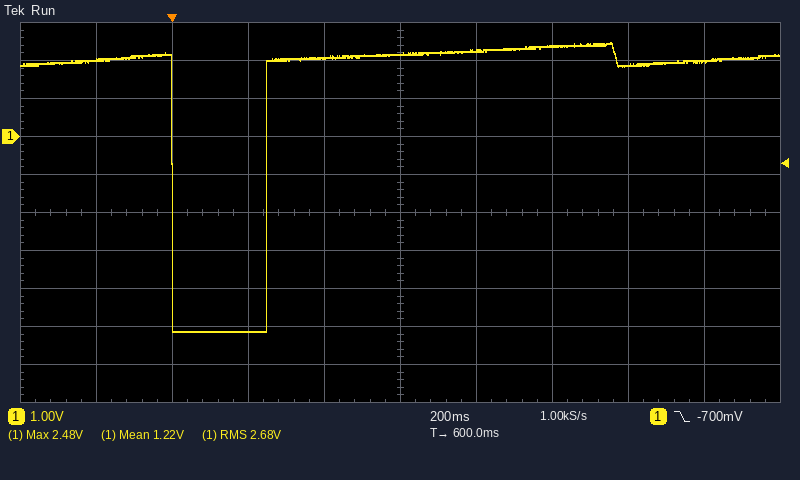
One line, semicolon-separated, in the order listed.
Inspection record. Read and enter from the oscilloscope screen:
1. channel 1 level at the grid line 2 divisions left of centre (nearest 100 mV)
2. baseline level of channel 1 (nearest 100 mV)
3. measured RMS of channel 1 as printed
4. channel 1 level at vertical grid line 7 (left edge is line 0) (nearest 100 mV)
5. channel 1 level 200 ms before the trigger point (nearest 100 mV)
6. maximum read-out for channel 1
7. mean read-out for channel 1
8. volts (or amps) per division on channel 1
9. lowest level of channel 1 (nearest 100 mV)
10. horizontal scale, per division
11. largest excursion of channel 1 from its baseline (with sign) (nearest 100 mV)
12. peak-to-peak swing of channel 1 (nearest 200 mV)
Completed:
-5.1 V; 2.1 V; 2.68 V; 2.4 V; 2.0 V; 2.48 V; 1.22 V; 1 V; -5.1 V; 200 ms; -7.2 V; 7.6 V
